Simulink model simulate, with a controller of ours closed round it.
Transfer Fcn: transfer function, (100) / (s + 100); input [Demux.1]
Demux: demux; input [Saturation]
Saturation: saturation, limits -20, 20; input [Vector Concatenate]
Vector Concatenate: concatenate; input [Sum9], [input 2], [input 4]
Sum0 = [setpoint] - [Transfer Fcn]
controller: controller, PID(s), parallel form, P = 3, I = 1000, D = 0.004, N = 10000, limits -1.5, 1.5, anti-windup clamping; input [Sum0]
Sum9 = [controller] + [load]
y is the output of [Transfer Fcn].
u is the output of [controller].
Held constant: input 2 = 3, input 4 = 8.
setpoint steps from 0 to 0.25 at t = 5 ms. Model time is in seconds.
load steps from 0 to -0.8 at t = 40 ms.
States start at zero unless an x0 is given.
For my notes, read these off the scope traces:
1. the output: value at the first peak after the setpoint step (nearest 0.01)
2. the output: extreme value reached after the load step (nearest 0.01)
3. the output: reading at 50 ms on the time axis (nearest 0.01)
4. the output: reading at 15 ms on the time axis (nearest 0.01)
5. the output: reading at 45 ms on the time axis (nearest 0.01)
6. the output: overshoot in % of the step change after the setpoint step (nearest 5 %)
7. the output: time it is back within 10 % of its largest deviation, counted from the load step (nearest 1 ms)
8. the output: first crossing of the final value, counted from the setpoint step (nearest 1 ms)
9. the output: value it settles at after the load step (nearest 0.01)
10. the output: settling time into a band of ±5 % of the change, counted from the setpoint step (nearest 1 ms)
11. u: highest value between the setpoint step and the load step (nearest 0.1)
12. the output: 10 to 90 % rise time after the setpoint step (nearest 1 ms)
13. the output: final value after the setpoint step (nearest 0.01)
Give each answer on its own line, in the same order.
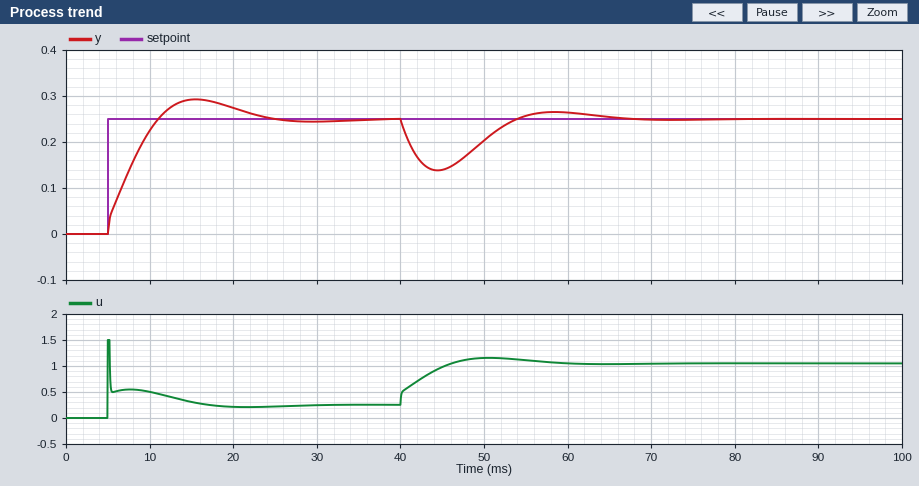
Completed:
0.29
0.14
0.20
0.29
0.14
15 %
22 ms
6 ms
0.25
17 ms
1.5
5 ms
0.25
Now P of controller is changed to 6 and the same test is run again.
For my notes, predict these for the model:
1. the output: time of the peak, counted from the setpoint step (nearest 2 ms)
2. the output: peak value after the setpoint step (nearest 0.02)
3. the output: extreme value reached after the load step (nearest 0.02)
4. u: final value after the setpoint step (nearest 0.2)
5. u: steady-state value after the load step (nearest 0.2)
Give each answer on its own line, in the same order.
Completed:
10 ms
0.26
0.16
0.2
1.0
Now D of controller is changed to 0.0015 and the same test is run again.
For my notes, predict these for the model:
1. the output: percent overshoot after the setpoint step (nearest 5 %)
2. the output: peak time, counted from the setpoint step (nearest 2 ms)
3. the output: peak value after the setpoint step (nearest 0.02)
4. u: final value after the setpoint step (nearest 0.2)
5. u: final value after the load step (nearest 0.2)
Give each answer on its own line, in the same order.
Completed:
15 %
10 ms
0.28
0.2
1.0
